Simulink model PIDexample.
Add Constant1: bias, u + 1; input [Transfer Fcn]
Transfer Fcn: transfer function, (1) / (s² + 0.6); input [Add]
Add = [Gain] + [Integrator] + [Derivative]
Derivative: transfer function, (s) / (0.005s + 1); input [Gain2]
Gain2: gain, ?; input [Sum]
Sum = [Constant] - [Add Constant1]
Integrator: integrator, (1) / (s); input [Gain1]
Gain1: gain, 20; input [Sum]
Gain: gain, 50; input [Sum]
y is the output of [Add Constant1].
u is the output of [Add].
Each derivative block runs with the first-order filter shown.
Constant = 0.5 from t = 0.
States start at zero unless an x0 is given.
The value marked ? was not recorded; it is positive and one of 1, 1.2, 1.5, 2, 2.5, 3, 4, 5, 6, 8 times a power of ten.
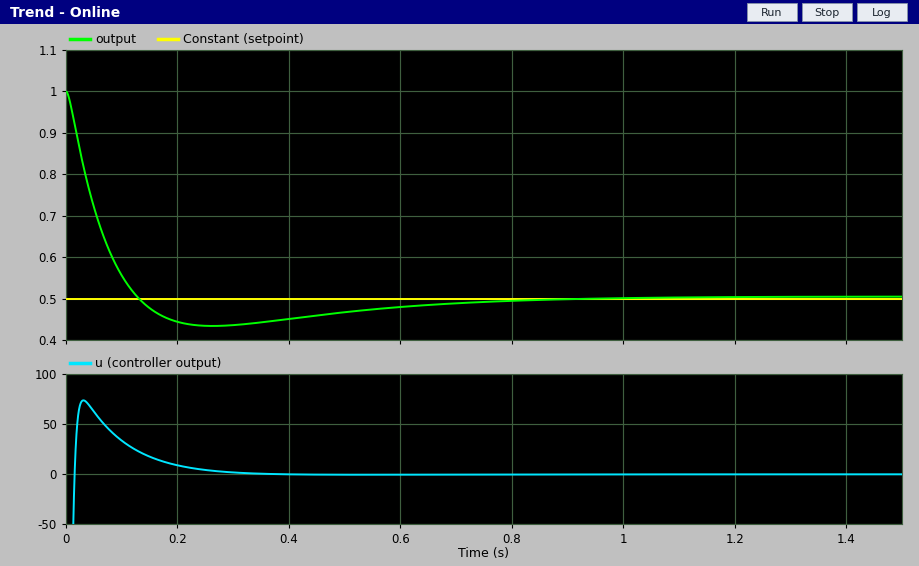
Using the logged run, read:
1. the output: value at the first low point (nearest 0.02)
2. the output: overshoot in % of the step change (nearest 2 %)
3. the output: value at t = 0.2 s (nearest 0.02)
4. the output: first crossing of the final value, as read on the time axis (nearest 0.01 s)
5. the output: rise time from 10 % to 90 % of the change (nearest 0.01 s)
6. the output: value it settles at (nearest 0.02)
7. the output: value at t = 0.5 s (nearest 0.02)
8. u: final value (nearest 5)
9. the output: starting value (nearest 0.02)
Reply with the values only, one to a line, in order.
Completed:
0.44
14 %
0.44
0.13 s
0.09 s
0.50
0.46
0
1.00
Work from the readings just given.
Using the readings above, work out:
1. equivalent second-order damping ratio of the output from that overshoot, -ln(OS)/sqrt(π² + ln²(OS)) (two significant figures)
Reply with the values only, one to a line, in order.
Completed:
0.53
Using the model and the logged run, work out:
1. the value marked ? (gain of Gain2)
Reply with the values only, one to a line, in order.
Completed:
15
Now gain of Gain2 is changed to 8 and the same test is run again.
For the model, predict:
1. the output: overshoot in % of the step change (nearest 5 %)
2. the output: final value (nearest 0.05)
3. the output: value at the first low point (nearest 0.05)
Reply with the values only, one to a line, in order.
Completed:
30 %
0.50
0.35
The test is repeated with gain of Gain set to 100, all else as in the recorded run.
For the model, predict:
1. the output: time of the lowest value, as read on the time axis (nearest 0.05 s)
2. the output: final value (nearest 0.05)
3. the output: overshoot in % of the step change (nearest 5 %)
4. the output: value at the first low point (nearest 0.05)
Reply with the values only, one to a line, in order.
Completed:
0.20 s
0.50
20 %
0.40
